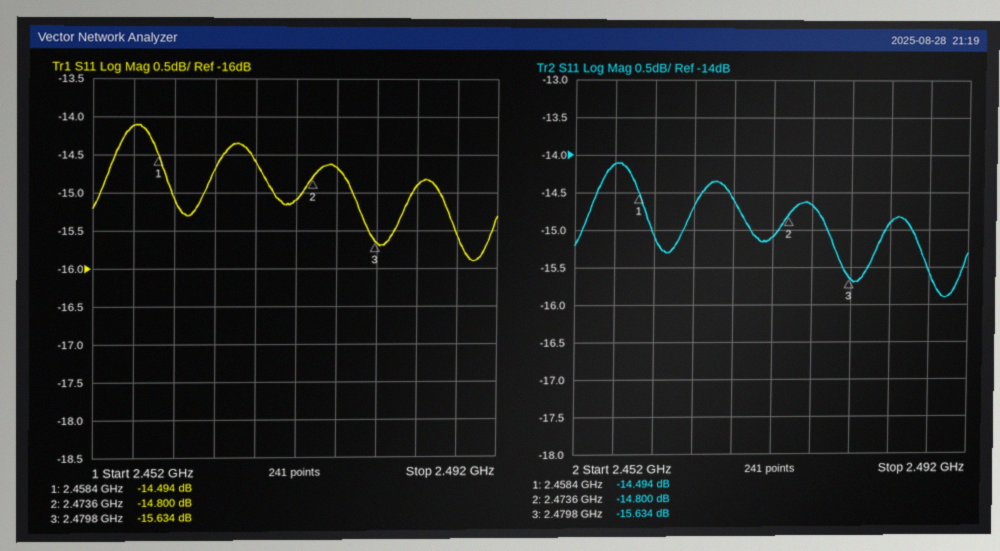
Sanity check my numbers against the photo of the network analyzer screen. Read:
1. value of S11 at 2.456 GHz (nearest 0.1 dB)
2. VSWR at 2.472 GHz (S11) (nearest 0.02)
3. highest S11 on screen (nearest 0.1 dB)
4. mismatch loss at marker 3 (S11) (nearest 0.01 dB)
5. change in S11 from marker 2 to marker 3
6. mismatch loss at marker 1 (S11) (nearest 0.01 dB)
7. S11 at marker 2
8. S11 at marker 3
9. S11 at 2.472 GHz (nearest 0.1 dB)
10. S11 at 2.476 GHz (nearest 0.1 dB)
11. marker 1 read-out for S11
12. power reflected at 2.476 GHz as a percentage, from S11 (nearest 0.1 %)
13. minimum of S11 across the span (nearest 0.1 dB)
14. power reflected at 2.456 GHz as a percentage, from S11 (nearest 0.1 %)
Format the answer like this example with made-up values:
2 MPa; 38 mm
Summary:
-14.1 dB; 1.42; -14.1 dB; 0.12 dB; -0.834 dB; 0.16 dB; -14.800 dB; -15.634 dB; -15.1 dB; -14.7 dB; -14.494 dB; 3.4 %; -15.9 dB; 3.9 %
